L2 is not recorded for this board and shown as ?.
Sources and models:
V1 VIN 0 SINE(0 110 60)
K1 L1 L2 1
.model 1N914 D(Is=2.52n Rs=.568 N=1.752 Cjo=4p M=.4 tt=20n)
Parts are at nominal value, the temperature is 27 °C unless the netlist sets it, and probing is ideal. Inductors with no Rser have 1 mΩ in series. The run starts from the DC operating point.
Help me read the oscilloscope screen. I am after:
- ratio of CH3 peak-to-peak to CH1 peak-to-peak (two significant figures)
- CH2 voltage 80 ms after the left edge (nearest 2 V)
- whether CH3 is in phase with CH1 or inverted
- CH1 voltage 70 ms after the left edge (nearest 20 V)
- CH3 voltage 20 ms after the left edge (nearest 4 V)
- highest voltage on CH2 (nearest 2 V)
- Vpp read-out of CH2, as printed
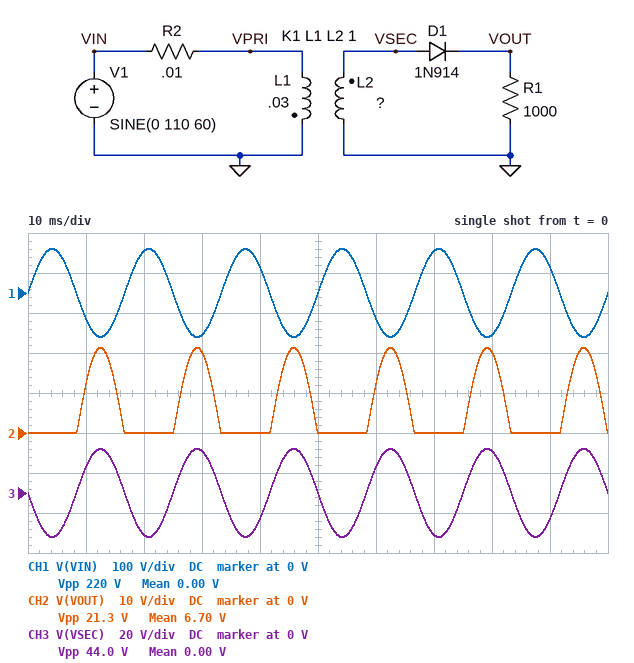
0.20
20 V
inverted
100 V
-20 V
22 V
21.3 V
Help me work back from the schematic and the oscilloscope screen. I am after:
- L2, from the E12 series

1.2 mH
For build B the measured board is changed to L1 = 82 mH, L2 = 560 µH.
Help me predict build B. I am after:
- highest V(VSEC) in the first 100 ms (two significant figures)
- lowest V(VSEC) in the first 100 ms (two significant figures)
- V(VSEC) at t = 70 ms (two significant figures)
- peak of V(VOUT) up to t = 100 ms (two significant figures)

9.1 V
-9.1 V
-8.6 V
8.4 V
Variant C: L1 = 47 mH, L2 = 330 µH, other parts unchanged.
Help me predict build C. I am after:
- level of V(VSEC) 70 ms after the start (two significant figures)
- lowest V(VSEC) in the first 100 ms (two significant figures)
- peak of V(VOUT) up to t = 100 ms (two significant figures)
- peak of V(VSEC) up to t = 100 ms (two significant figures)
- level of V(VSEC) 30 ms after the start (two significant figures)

-8.8 V
-9.2 V
8.5 V
9.2 V
8.8 V
